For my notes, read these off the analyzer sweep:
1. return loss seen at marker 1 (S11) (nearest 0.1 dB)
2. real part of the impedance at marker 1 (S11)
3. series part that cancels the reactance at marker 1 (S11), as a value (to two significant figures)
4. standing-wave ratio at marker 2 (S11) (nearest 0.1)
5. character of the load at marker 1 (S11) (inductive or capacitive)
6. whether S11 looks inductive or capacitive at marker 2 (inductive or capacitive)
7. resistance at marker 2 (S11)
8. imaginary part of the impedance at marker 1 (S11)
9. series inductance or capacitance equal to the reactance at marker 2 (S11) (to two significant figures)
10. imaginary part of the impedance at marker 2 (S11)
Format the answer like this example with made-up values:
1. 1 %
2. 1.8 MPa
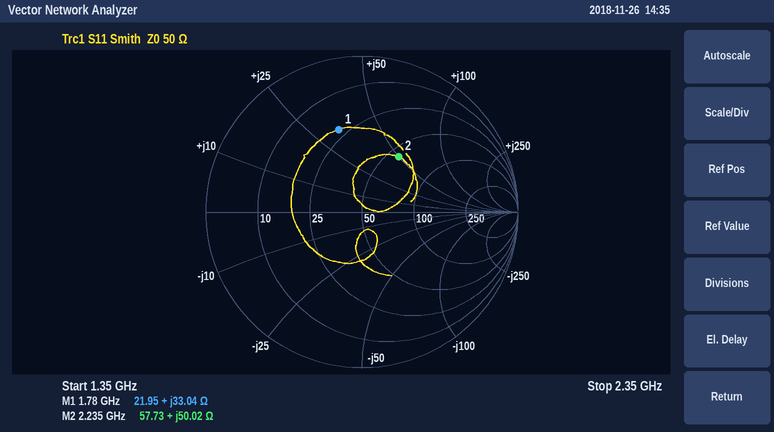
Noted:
1. 5.2 dB
2. 21.95 Ω
3. 2.7 pF
4. 2.5
5. inductive
6. inductive
7. 57.73 Ω
8. +33.04 Ω
9. 3.6 nH
10. +50.02 Ω
